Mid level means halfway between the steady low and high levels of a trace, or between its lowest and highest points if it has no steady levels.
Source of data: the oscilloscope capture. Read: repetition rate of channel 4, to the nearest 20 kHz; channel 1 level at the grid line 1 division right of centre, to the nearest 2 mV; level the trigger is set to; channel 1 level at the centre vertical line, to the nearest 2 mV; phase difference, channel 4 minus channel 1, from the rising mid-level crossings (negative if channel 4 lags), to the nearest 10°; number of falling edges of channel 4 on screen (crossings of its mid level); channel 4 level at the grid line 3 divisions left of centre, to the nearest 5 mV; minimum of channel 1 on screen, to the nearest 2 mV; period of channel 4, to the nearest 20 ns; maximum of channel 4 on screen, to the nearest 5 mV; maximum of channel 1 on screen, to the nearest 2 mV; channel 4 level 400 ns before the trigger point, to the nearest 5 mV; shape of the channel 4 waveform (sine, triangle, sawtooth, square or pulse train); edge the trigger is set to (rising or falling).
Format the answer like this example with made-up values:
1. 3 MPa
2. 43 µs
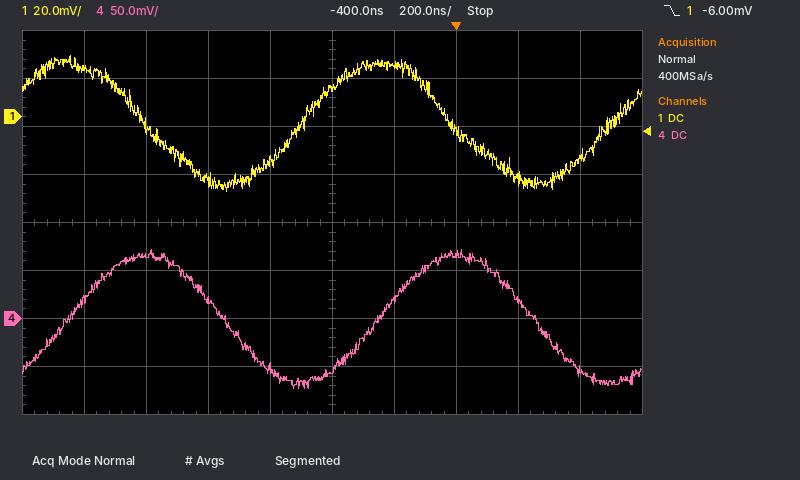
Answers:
1. 1.00 MHz
2. 22 mV
3. -6.00 mV
4. 12 mV
5. -90°
6. 2
7. 65 mV
8. -32 mV
9. 1.00 µs
10. 70 mV
11. 26 mV
12. -55 mV
13. sine
14. falling
